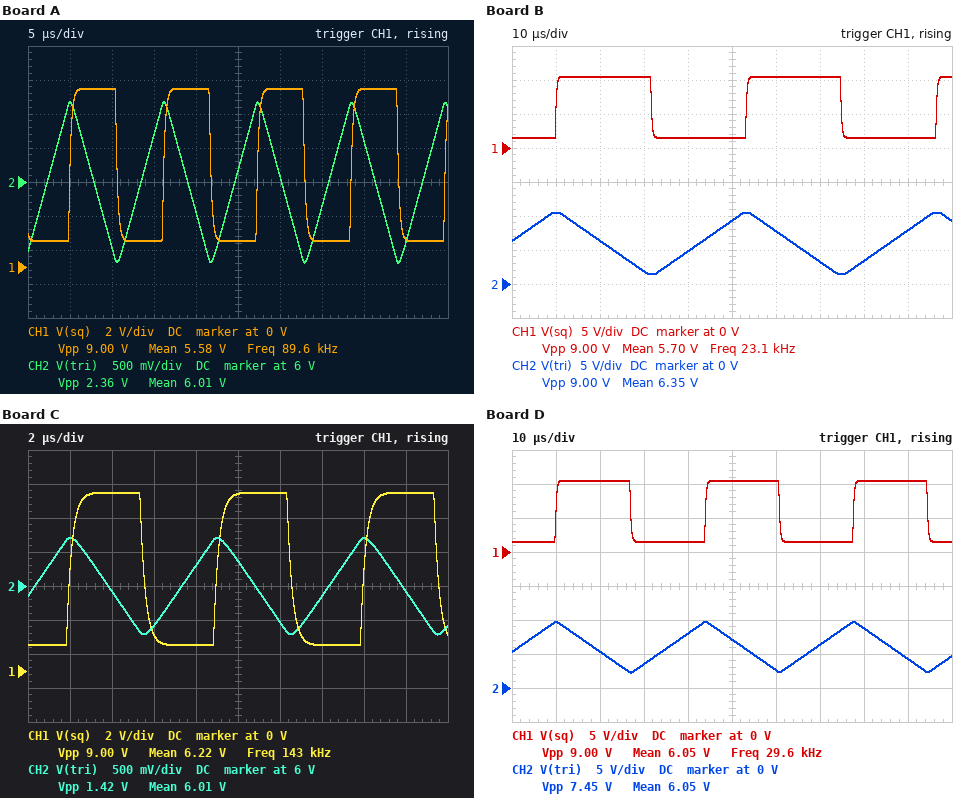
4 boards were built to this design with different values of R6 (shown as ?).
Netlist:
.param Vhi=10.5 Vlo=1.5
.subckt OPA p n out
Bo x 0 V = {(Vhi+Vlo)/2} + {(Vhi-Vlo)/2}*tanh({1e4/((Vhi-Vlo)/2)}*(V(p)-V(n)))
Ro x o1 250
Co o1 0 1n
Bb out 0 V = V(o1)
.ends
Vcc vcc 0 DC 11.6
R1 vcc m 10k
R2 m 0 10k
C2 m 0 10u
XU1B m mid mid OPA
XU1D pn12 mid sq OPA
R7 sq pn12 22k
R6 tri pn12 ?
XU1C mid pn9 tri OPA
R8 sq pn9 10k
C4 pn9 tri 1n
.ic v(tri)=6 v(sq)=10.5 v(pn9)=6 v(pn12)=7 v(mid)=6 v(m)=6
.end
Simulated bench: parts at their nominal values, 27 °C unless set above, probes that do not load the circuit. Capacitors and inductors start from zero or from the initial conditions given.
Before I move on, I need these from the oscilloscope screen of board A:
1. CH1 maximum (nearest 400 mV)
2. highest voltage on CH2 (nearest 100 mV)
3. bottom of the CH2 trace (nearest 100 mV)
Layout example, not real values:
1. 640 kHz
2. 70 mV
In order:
1. 10.4 V
2. 7.2 V
3. 4.8 V
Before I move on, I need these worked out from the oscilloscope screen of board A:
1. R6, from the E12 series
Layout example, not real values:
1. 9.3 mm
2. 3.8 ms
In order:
1. 5.6 kΩ
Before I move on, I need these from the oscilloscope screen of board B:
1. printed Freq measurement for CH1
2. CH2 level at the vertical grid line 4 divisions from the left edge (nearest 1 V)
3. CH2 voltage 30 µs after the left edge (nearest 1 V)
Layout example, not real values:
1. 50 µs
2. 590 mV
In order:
1. 23.1 kHz
2. 5 V
3. 2 V
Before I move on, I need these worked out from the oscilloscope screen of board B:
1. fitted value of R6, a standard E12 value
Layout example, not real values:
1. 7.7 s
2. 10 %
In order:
1. 22 kΩ
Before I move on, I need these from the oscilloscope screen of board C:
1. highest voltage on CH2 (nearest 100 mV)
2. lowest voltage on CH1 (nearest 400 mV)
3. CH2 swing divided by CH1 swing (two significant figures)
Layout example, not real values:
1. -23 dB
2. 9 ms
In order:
1. 6.7 V
2. 1.6 V
3. 0.16
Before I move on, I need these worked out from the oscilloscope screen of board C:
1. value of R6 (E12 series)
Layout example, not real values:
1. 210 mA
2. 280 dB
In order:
1. 3.3 kΩ
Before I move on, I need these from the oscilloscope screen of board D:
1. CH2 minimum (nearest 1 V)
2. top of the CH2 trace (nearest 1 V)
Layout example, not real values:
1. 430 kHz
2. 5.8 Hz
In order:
1. 2 V
2. 10 V
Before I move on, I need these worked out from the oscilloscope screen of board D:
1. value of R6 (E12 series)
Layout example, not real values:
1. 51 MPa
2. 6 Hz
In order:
1. 18 kΩ
